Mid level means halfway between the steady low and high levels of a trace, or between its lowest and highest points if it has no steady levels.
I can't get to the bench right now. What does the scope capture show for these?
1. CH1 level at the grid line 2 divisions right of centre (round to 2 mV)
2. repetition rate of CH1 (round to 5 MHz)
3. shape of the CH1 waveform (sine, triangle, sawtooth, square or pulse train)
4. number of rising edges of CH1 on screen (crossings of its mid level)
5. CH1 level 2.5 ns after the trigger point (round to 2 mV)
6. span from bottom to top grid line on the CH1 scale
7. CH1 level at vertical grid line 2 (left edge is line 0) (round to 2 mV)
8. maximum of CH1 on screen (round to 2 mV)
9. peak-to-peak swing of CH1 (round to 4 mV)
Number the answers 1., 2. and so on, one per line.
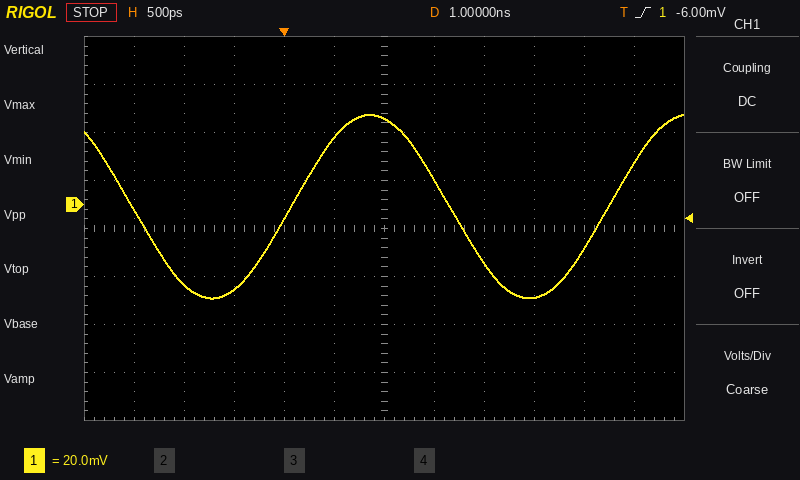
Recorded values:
1. -24 mV
2. 315 MHz
3. sine
4. 2
5. -38 mV
6. 160 mV
7. -34 mV
8. 38 mV
9. 76 mV
